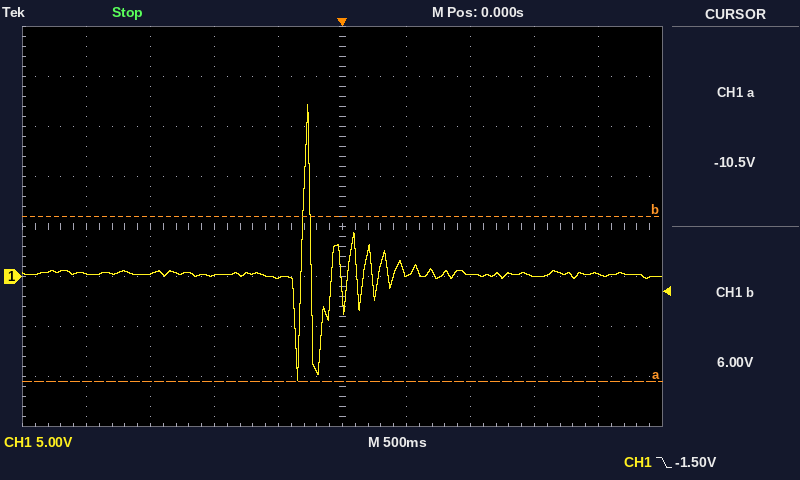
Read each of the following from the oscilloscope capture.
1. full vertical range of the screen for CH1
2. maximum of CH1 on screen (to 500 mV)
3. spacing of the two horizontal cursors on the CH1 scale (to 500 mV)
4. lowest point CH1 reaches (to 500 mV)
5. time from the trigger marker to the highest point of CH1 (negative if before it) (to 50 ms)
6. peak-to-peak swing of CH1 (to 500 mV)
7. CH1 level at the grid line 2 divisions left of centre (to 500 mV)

40 V
17.0 V
16.5 V
-10.5 V
-250 ms
27.5 V
0.0 V
